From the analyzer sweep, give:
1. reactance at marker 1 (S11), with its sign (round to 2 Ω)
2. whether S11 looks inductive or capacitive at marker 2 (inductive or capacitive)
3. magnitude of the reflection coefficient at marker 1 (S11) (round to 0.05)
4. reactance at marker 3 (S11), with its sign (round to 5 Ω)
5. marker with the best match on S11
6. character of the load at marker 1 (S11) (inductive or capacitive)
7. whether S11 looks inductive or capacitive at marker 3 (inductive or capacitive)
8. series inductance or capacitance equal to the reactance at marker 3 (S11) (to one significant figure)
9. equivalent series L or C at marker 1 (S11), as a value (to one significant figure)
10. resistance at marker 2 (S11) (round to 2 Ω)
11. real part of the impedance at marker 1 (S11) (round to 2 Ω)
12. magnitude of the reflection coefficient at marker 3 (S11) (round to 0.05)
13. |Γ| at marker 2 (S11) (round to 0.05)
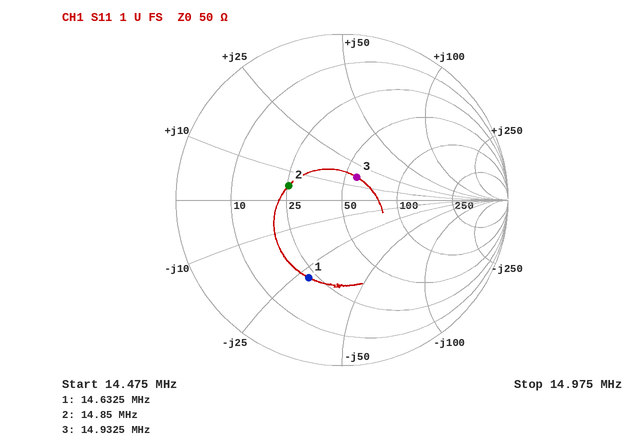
-28 Ω
inductive
0.50
+15 Ω
marker 3
capacitive
inductive
200 nH
400 pF
26 Ω
22 Ω
0.15
0.35
